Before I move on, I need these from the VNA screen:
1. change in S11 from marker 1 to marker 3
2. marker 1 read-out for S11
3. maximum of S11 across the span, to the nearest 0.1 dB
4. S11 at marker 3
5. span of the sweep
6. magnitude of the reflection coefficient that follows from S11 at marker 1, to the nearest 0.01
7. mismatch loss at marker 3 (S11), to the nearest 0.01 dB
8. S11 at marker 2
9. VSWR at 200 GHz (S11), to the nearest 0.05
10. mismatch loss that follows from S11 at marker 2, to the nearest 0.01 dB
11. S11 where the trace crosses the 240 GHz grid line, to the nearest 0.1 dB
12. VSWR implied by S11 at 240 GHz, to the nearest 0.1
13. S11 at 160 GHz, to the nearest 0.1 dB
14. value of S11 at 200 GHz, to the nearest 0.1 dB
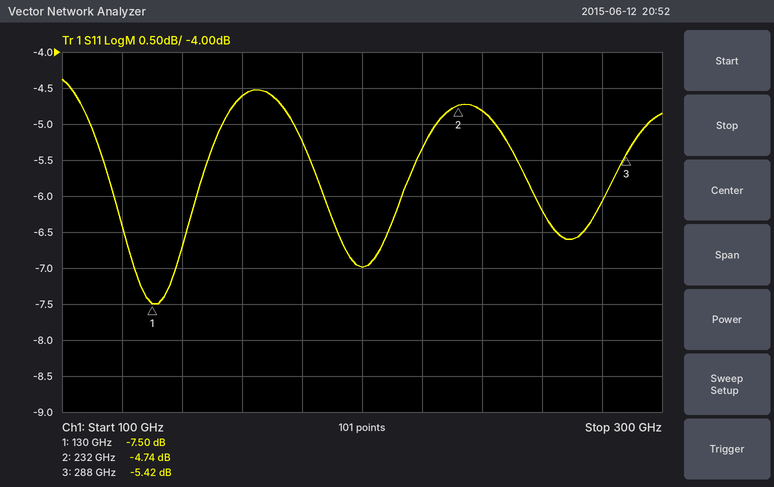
2.08 dB
-7.50 dB
-4.4 dB
-5.42 dB
200 GHz
0.42
1.47 dB
-4.74 dB
2.60
1.78 dB
-4.8 dB
3.7
-4.6 dB
-7.0 dB
